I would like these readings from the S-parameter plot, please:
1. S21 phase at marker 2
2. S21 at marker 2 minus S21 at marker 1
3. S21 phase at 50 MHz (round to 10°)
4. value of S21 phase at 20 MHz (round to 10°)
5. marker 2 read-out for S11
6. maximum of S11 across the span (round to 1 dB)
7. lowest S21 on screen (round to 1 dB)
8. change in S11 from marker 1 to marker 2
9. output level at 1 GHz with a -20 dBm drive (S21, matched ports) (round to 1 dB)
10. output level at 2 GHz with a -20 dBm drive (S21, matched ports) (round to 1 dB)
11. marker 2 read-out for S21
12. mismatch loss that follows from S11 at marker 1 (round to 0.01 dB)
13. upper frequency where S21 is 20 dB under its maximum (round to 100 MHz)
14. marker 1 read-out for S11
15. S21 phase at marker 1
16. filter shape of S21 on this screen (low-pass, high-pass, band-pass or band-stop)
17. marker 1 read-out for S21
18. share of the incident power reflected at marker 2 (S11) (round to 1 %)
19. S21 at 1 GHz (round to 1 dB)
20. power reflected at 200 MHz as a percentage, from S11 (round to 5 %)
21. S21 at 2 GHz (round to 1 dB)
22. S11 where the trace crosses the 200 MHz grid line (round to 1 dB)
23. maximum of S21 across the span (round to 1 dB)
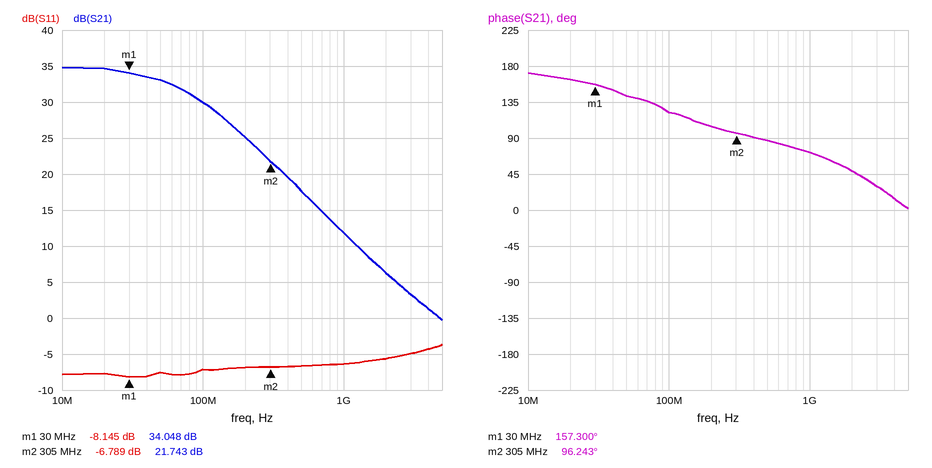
96.243°
-12.305 dB
140°
160°
-6.789 dB
-4 dB
0 dB
1.356 dB
-8 dBm
-14 dBm
21.743 dB
0.72 dB
700 MHz
-8.145 dB
157.300°
low-pass
34.048 dB
21 %
12 dB
20 %
6 dB
-7 dB
35 dB
